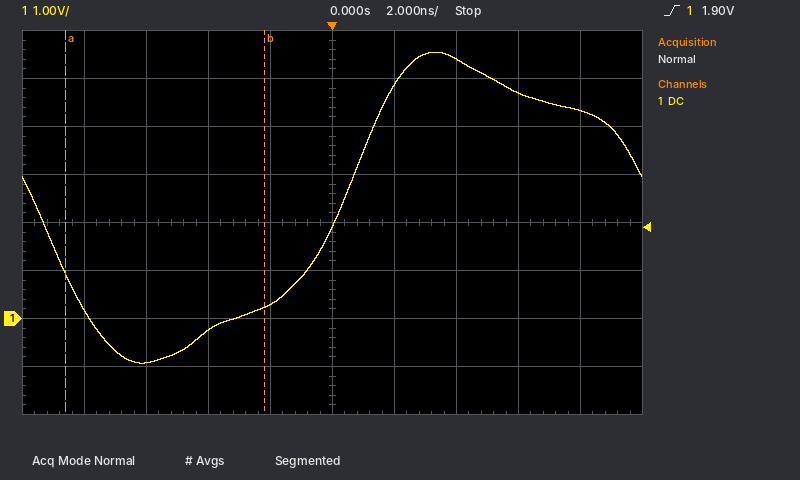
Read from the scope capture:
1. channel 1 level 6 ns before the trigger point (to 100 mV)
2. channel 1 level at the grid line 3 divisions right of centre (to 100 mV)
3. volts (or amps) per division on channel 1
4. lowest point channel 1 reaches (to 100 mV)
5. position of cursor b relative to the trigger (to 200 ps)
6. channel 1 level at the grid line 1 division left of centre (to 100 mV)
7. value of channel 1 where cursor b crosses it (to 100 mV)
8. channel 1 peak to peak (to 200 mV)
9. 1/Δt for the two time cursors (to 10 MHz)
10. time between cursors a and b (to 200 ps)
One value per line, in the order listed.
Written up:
-900 mV
4.7 V
1 V
-900 mV
-2.2 ns
300 mV
200 mV
6.4 V
160 MHz
6.4 ns
